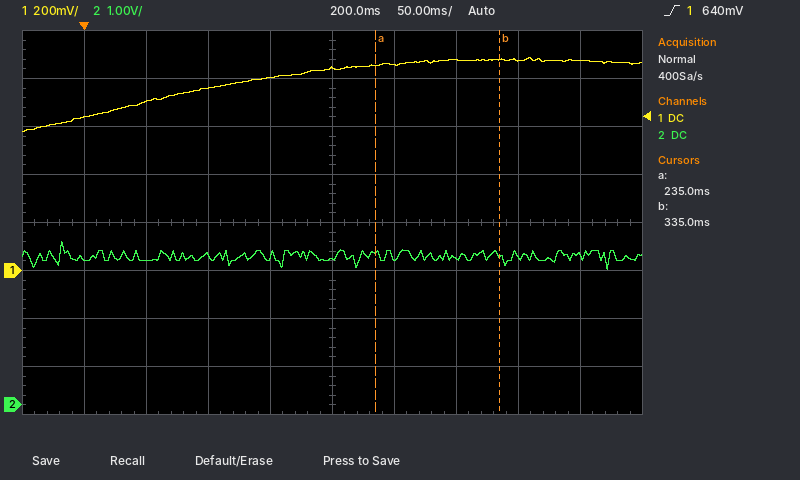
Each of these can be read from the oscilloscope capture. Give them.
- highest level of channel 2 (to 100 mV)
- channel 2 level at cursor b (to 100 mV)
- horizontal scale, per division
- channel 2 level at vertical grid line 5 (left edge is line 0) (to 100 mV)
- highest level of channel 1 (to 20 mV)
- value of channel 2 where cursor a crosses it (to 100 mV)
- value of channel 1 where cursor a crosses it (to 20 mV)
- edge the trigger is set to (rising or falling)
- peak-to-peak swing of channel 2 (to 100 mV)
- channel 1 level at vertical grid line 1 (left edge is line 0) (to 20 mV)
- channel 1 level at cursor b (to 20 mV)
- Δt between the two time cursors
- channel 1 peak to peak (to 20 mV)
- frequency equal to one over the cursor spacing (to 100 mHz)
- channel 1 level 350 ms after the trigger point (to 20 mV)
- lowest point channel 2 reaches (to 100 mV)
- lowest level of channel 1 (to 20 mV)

3.4 V
3.1 V
50 ms
3.0 V
880 mV
3.2 V
860 mV
rising
600 mV
640 mV
880 mV
100 ms
300 mV
10.0 Hz
880 mV
2.8 V
580 mV
